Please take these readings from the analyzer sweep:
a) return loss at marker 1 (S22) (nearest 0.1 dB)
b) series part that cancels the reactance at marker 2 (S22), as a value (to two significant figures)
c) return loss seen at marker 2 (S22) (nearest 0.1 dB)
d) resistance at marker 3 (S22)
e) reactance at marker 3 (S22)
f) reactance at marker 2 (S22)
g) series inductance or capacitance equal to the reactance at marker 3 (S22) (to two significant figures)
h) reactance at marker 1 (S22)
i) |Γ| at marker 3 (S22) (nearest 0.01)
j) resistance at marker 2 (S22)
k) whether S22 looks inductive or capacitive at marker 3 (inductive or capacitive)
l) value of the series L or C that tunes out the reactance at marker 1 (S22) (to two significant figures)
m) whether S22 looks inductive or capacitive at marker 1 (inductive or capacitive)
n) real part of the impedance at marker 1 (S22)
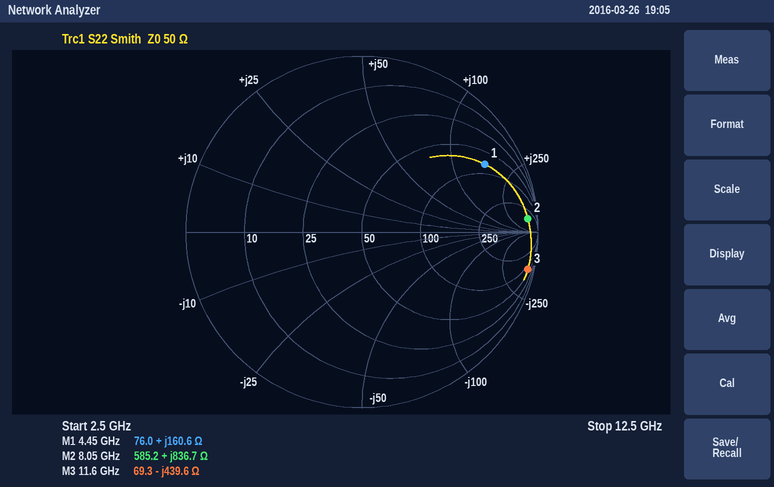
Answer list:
2.0 dB
24 fF
0.5 dB
69.3 Ω
-439.6 Ω
+836.7 Ω
31 fF
+160.6 Ω
0.97
585.2 Ω
capacitive
220 fF
inductive
76.0 Ω
